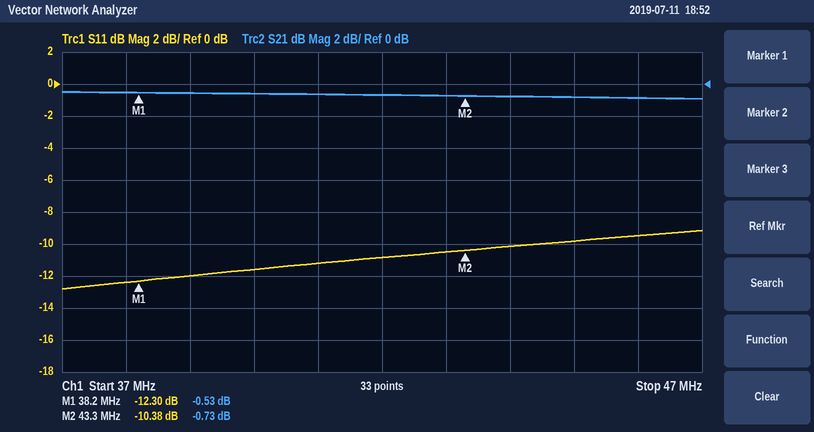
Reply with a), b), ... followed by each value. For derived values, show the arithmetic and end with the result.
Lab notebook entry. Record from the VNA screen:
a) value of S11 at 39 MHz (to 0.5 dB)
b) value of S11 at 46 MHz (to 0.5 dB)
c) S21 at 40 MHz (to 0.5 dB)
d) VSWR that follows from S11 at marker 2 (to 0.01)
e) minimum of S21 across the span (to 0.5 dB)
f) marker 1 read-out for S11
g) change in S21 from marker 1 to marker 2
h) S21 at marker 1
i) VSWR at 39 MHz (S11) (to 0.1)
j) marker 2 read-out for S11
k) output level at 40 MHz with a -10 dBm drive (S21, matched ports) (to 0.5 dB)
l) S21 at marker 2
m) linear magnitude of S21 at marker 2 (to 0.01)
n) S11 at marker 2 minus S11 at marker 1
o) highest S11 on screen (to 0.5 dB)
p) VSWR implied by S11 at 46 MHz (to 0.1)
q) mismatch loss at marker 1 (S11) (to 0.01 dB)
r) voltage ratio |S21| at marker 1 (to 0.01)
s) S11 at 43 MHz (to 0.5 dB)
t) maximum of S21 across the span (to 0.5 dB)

a) -12.0 dB
b) -9.5 dB
c) -0.5 dB
d) (1 + 0.3027)/(1 − 0.3027) ≈ 1.87
e) -1.0 dB
f) -12.30 dB
g) -0.73 − (-0.53) = -0.20 dB
h) -0.53 dB
i) |Γ| = 10^(-12/20) = 0.2512; VSWR = (1 + 0.2512)/(1 − 0.2512) ≈ 1.7
j) -10.38 dB
k) -10 dBm + (-0.5 dB) = -10.5 dBm
l) -0.73 dB
m) 10^(-0.73/20) ≈ 0.92
n) -10.38 − (-12.3) = 1.92 dB
o) -9.0 dB
p) |Γ| = 10^(-9.5/20) = 0.3350; VSWR = (1 + 0.3350)/(1 − 0.3350) ≈ 2.0
q) −10 log10(1 − 10^(-12.3/10)) ≈ 0.26 dB
r) 10^(-0.53/20) ≈ 0.94
s) -10.5 dB
t) -0.5 dB
